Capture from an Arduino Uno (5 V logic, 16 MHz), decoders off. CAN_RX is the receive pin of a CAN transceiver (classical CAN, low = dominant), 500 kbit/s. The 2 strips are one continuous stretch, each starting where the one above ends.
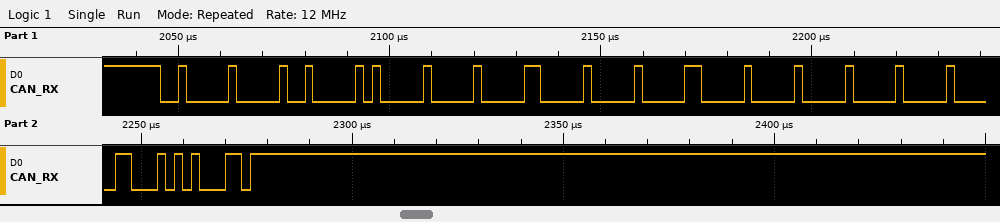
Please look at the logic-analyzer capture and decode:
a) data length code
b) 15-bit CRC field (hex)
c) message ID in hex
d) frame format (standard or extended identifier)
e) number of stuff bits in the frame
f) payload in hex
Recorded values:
8
0x1151
0x200
standard
15
10 00 10 00 10 00 00 00
